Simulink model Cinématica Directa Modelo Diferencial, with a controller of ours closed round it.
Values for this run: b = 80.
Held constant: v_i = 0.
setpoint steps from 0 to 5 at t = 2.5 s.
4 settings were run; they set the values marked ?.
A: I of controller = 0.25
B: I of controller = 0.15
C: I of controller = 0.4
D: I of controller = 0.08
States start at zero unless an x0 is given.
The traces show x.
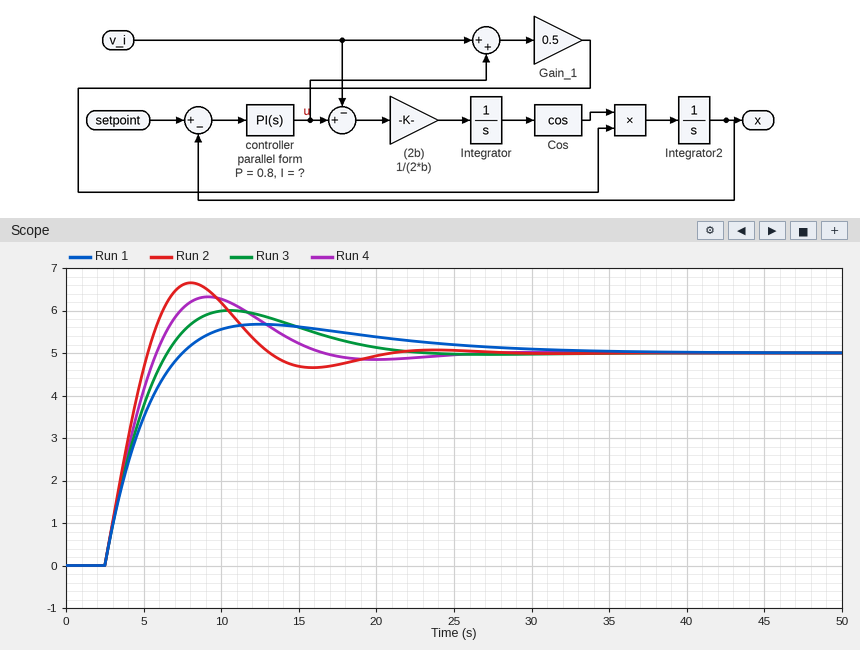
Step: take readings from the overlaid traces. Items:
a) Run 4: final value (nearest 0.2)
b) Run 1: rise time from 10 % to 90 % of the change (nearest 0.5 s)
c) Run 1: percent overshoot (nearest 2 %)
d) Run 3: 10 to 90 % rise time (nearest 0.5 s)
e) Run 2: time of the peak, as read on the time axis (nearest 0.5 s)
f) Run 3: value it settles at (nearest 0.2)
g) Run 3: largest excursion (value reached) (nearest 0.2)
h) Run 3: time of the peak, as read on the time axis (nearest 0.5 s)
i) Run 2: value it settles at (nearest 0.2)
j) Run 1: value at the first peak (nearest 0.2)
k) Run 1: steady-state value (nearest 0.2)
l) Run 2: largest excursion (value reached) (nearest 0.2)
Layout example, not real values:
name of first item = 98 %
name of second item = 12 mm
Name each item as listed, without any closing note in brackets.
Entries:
Run 4: final value = 5.0
Run 1: rise time from 10 % to 90 % of the change = 3.5 s
Run 1: percent overshoot = 14 %
Run 3: 10 to 90 % rise time = 3.0 s
Run 2: time of the peak, as read on the time axis = 8.0 s
Run 3: value it settles at = 5.0
Run 3: largest excursion (value reached) = 6.0
Run 3: time of the peak, as read on the time axis = 10.5 s
Run 2: value it settles at = 5.0
Run 1: value at the first peak = 5.6
Run 1: steady-state value = 5.0
Run 2: largest excursion (value reached) = 6.6
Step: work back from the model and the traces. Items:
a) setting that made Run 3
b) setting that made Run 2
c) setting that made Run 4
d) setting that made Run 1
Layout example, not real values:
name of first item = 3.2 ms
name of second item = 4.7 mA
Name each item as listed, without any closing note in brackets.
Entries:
setting that made Run 3 = B
setting that made Run 2 = C
setting that made Run 4 = A
setting that made Run 1 = D
